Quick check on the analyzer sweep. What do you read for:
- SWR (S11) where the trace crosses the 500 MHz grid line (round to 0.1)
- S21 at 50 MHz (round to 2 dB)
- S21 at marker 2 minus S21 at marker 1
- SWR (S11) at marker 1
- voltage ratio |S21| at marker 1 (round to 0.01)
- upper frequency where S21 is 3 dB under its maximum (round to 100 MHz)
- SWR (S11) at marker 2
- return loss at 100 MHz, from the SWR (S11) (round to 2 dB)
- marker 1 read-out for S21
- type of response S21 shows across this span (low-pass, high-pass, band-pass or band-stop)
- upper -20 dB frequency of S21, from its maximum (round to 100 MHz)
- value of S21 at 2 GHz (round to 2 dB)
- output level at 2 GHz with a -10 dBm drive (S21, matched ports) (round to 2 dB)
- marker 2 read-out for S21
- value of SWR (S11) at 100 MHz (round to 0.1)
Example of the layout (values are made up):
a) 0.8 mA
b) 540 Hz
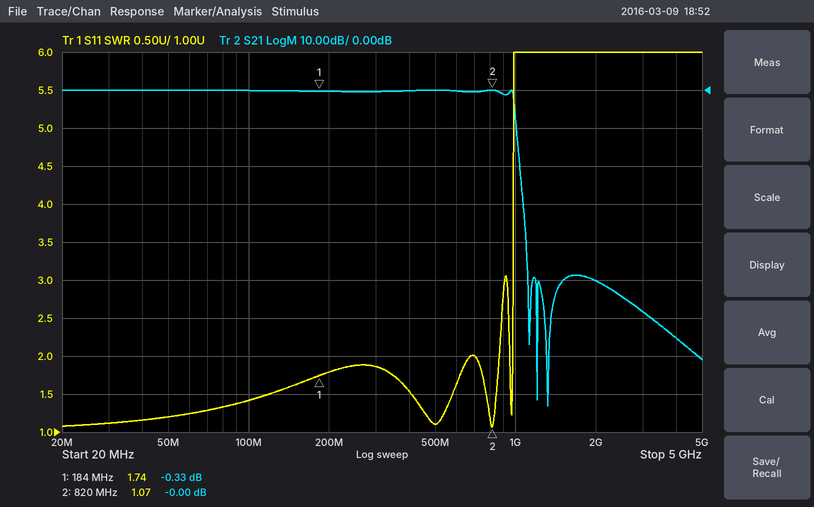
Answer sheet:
a) 1.1
b) 0 dB
c) 0.33 dB
d) 1.74
e) 0.96
f) 1.0 GHz
g) 1.07
h) 16 dB
i) -0.33 dB
j) low-pass
k) 1.0 GHz
l) -50 dB
m) -60 dBm
n) -0.00 dB
o) 1.4
